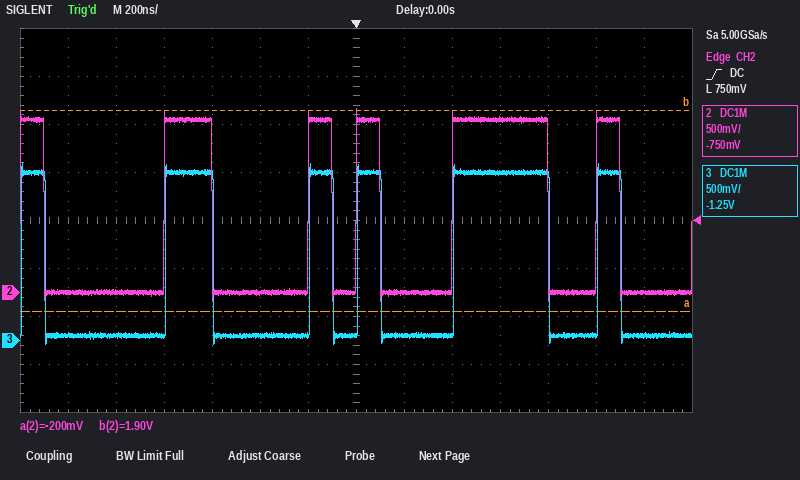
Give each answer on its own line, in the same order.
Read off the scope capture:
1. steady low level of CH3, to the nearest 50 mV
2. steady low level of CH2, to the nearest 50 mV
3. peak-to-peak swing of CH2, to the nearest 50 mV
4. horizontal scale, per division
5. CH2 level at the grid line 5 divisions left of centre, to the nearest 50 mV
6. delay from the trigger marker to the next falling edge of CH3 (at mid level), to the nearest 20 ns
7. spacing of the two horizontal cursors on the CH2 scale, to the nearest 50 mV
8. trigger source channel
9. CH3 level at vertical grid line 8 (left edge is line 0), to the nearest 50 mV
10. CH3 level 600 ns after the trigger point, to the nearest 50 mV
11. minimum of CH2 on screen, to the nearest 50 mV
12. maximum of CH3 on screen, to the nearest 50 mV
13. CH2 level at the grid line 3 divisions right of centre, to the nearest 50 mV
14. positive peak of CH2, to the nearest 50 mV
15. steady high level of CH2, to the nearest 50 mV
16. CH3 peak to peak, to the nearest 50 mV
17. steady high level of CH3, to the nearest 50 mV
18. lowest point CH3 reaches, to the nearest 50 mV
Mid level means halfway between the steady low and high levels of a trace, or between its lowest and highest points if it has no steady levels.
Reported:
50 mV
0 mV
2.00 V
200 ns
0 mV
100 ns
2.10 V
CH2
50 mV
1.75 V
-100 mV
1.85 V
1.80 V
1.90 V
1.80 V
1.90 V
1.75 V
-50 mV
